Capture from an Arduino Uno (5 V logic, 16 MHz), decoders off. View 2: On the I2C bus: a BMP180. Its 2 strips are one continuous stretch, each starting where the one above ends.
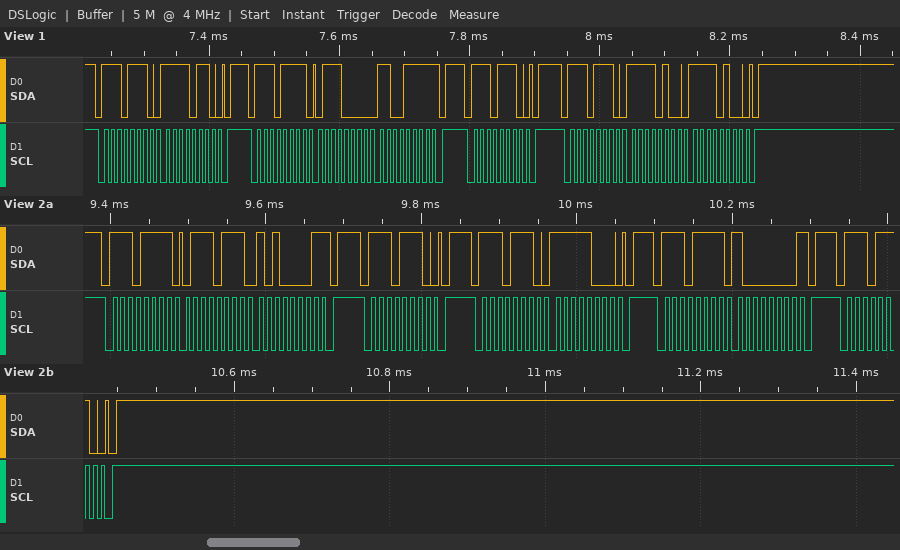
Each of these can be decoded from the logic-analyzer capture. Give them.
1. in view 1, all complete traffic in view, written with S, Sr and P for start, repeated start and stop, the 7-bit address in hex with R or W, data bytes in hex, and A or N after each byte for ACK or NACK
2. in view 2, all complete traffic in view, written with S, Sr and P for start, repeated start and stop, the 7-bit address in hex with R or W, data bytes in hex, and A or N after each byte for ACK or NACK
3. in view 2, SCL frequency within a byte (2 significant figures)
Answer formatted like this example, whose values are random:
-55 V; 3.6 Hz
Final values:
S 77W A F6 A P S 77R A 70 A CF N P S 77W A P S 77W A F4 A F4 A P; S 77R A 77 A A1 N P S 77W A P S 77W A F8 A P S 77R A 80 N P S 77W A P; 100 kHz
